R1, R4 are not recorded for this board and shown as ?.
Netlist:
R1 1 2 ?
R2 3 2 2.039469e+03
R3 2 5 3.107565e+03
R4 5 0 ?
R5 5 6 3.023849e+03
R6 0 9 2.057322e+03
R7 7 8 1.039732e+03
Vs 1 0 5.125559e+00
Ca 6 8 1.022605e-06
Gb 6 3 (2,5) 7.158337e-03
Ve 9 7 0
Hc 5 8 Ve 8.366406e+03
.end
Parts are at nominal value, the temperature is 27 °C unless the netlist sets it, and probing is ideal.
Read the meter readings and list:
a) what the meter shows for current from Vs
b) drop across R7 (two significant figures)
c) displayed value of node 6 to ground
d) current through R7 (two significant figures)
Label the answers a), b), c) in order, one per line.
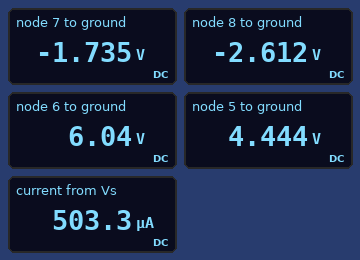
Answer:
a) 503.3 µA
b) 880 mV
c) 6.04 V
d) 840 µA
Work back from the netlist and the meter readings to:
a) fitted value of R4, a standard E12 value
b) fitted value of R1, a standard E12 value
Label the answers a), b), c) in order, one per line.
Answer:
a) 3.3 kΩ
b) 1.5 kΩ
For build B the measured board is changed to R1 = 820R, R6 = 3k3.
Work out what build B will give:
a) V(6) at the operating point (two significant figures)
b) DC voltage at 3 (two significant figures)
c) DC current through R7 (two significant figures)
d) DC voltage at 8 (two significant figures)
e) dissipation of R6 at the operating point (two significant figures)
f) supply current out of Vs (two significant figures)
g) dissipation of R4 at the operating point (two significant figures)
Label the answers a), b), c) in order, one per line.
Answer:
a) 5.8 V
b) 4.3 V
c) 1.2 mA
d) -5.3 V
e) 5.0 mW
f) 270 µA
g) 7.4 mW
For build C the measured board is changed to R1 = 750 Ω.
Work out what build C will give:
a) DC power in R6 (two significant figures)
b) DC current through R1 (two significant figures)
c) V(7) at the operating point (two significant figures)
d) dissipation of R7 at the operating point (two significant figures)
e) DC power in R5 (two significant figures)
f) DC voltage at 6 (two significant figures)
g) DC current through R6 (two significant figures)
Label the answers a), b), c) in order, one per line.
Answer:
a) 1.7 mW
b) 540 µA
c) -1.9 V
d) 860 µW
e) 980 µW
f) 6.5 V
g) 910 µA
